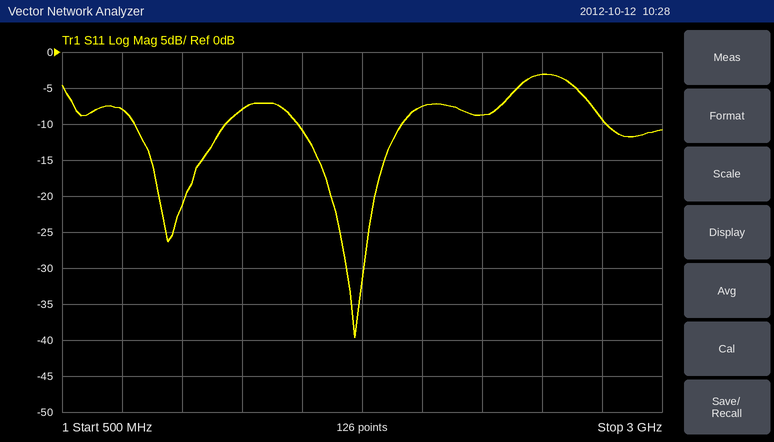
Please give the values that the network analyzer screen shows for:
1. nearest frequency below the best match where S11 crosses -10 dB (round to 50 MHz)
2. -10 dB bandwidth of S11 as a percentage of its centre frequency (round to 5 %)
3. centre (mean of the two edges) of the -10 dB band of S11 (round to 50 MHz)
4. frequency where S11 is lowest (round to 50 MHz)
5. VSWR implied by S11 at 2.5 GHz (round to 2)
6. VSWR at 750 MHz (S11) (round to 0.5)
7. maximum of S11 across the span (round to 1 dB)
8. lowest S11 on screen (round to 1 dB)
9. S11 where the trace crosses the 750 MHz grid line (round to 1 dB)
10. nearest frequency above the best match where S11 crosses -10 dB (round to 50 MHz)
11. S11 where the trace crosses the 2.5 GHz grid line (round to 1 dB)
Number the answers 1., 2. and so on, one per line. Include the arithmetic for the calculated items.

1. 1.50 GHz
2. 400 MHz / 1.7 GHz ≈ 23.5 %, so 25 % to the nearest 5 %
3. 1.70 GHz
4. 1.70 GHz
5. |Γ| = 10^(-3/20) = 0.7079; VSWR = (1 + 0.7079)/(1 − 0.7079) ≈ 6
6. |Γ| = 10^(-8/20) = 0.3981; VSWR = (1 + 0.3981)/(1 − 0.3981) ≈ 2.32, so 2.5 to the nearest 0.5
7. -3 dB
8. -40 dB
9. -8 dB
10. 1.90 GHz
11. -3 dB
